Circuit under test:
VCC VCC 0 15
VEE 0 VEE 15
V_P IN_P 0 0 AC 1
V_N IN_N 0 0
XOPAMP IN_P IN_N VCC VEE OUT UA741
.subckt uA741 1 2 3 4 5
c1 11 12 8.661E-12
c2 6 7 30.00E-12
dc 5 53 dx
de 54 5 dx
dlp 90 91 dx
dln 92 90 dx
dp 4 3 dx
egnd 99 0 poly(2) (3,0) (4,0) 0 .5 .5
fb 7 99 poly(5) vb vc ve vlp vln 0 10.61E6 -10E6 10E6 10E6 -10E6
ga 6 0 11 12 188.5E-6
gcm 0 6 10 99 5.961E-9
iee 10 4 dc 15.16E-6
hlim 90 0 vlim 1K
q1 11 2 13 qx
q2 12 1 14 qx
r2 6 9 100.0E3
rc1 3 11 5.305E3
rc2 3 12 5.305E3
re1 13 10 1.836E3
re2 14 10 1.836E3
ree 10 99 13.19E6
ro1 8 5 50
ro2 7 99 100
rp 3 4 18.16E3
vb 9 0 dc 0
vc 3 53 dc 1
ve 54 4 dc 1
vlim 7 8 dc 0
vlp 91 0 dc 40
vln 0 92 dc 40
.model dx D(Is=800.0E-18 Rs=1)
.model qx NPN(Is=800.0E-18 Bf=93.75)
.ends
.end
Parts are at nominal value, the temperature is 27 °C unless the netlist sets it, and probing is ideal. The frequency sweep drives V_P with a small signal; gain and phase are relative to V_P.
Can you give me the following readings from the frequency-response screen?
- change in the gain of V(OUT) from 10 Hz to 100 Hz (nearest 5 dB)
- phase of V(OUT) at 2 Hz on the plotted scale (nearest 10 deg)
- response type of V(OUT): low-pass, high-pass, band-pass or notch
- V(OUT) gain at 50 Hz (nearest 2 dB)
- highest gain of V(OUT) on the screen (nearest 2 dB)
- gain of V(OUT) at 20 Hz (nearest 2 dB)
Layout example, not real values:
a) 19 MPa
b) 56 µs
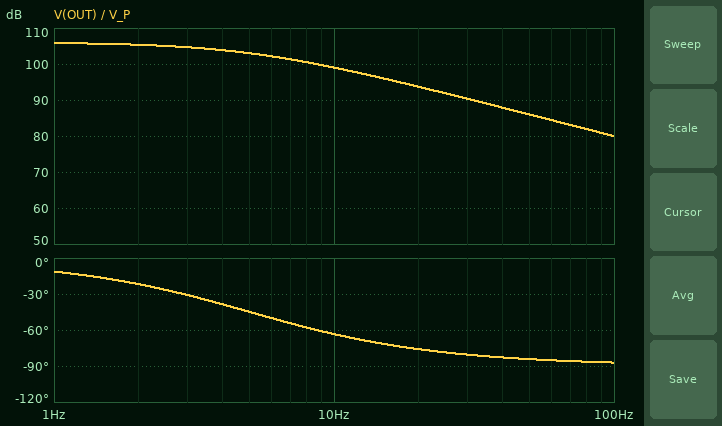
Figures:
a) -20 dB
b) -20 deg
c) low-pass
d) 86 dB
e) 106 dB
f) 94 dB
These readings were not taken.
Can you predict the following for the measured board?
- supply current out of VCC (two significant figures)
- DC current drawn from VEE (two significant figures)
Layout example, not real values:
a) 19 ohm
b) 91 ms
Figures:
a) 1.7 mA
b) 1.7 mA
